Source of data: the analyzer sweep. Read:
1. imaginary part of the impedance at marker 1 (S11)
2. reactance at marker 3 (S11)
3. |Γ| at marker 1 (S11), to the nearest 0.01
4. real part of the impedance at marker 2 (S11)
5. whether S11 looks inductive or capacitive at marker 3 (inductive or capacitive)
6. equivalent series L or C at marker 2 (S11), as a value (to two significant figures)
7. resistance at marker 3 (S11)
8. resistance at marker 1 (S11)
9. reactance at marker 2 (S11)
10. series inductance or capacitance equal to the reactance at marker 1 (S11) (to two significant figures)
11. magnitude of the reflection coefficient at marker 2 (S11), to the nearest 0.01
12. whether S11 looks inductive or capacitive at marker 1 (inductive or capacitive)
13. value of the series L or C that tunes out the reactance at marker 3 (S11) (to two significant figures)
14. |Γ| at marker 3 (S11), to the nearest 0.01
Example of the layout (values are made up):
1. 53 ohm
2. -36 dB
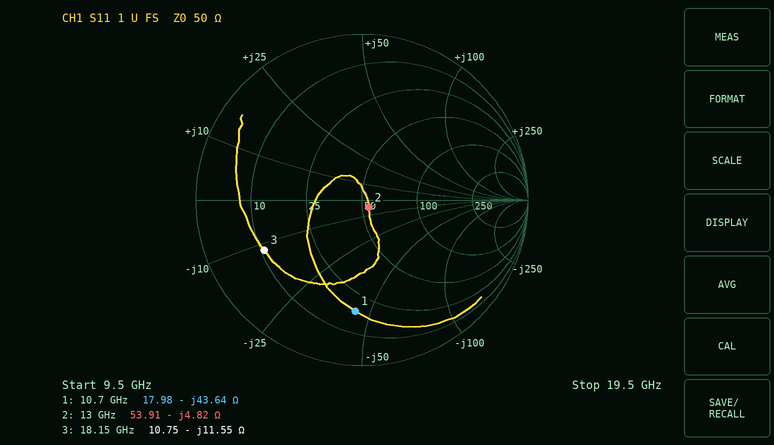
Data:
1. -43.64 Ω
2. -11.55 Ω
3. 0.67
4. 53.91 Ω
5. capacitive
6. 2.5 pF
7. 10.75 Ω
8. 17.98 Ω
9. -4.82 Ω
10. 340 fF
11. 0.06
12. capacitive
13. 100 pH
14. 0.66
